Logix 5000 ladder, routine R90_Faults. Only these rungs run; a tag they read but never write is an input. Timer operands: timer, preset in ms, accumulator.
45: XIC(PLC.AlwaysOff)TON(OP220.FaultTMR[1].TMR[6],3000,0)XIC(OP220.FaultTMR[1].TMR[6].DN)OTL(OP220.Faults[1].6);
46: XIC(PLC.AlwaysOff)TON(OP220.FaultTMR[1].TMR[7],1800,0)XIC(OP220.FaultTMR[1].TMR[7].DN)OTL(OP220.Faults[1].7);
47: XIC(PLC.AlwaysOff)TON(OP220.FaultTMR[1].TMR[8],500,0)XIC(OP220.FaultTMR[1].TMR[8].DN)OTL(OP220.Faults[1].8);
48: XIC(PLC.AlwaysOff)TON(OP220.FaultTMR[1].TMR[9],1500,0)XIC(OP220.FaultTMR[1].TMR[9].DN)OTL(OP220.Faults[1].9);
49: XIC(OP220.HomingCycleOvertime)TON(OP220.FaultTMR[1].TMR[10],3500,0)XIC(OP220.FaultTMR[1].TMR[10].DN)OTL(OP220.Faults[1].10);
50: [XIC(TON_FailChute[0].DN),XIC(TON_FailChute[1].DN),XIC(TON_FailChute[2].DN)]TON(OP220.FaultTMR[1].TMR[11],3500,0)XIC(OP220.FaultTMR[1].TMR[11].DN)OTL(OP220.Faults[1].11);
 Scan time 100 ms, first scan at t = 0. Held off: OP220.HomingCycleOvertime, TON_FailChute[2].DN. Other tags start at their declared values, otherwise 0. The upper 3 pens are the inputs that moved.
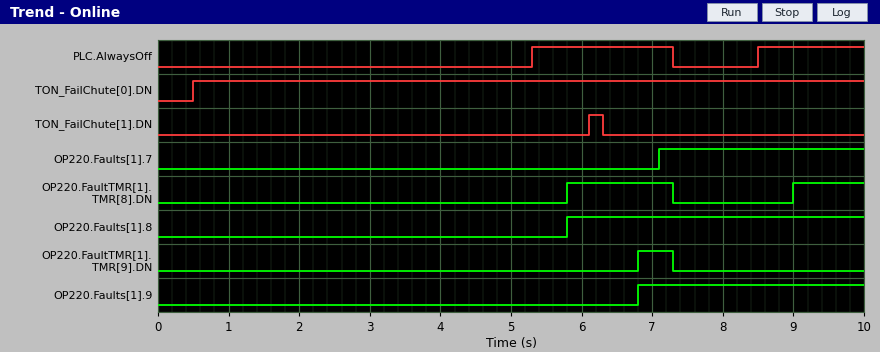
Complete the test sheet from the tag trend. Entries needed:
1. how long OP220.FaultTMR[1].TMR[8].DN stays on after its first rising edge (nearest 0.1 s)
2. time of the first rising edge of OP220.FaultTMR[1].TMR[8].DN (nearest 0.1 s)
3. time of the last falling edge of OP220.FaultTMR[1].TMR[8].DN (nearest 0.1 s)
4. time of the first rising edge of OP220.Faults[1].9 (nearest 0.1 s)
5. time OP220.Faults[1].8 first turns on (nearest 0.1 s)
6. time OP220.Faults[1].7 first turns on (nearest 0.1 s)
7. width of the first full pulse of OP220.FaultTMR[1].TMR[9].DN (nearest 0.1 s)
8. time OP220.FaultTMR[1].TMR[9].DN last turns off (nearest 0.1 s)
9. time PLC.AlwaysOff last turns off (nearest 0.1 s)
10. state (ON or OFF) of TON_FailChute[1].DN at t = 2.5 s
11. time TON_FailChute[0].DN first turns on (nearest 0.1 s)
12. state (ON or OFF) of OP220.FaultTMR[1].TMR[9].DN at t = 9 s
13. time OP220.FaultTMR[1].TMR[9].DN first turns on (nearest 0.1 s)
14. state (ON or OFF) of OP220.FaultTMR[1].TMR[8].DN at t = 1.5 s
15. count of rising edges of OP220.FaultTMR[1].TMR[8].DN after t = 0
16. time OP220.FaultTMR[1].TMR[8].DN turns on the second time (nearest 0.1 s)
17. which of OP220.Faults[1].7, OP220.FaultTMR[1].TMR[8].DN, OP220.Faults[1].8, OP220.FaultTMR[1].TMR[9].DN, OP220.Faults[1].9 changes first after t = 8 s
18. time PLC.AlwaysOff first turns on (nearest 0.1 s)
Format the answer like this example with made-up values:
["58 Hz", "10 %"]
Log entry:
["1.5 s", "5.8 s", "7.3 s", "6.8 s", "5.8 s", "7.1 s", "0.5 s", "7.3 s", "7.3 s", "OFF", "0.5 s", "OFF", "6.8 s", "OFF", "2", "9.0 s", "OP220.FaultTMR[1].TMR[8].DN", "5.3 s"]
